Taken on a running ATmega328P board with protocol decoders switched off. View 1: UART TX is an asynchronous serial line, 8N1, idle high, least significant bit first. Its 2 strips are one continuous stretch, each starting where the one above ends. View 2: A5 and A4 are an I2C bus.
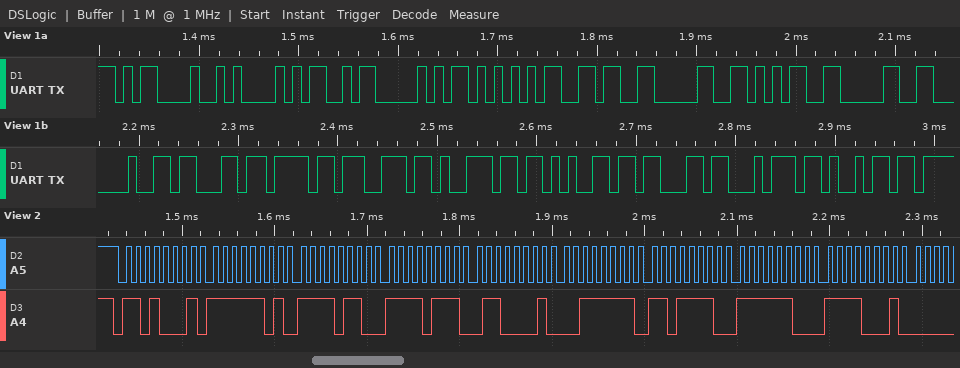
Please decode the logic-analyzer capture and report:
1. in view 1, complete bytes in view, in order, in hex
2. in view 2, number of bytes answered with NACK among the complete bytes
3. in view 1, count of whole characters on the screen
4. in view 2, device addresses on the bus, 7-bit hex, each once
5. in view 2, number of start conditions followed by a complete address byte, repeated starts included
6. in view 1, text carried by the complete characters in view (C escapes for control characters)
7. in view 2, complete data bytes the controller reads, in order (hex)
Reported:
0D 0A 4D 50 55 36 30 35 30 20 63 6F 6E 6E 65 63 74 69
0
18
0x68
1
"\r\nMPU6050 connecti"
FD F6 F7 61 3F DE FC F1
